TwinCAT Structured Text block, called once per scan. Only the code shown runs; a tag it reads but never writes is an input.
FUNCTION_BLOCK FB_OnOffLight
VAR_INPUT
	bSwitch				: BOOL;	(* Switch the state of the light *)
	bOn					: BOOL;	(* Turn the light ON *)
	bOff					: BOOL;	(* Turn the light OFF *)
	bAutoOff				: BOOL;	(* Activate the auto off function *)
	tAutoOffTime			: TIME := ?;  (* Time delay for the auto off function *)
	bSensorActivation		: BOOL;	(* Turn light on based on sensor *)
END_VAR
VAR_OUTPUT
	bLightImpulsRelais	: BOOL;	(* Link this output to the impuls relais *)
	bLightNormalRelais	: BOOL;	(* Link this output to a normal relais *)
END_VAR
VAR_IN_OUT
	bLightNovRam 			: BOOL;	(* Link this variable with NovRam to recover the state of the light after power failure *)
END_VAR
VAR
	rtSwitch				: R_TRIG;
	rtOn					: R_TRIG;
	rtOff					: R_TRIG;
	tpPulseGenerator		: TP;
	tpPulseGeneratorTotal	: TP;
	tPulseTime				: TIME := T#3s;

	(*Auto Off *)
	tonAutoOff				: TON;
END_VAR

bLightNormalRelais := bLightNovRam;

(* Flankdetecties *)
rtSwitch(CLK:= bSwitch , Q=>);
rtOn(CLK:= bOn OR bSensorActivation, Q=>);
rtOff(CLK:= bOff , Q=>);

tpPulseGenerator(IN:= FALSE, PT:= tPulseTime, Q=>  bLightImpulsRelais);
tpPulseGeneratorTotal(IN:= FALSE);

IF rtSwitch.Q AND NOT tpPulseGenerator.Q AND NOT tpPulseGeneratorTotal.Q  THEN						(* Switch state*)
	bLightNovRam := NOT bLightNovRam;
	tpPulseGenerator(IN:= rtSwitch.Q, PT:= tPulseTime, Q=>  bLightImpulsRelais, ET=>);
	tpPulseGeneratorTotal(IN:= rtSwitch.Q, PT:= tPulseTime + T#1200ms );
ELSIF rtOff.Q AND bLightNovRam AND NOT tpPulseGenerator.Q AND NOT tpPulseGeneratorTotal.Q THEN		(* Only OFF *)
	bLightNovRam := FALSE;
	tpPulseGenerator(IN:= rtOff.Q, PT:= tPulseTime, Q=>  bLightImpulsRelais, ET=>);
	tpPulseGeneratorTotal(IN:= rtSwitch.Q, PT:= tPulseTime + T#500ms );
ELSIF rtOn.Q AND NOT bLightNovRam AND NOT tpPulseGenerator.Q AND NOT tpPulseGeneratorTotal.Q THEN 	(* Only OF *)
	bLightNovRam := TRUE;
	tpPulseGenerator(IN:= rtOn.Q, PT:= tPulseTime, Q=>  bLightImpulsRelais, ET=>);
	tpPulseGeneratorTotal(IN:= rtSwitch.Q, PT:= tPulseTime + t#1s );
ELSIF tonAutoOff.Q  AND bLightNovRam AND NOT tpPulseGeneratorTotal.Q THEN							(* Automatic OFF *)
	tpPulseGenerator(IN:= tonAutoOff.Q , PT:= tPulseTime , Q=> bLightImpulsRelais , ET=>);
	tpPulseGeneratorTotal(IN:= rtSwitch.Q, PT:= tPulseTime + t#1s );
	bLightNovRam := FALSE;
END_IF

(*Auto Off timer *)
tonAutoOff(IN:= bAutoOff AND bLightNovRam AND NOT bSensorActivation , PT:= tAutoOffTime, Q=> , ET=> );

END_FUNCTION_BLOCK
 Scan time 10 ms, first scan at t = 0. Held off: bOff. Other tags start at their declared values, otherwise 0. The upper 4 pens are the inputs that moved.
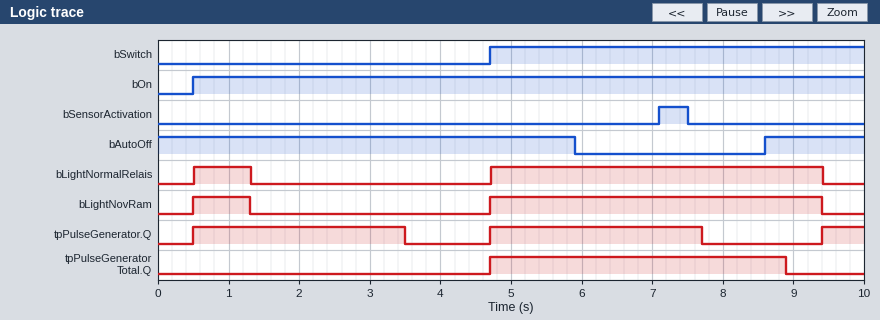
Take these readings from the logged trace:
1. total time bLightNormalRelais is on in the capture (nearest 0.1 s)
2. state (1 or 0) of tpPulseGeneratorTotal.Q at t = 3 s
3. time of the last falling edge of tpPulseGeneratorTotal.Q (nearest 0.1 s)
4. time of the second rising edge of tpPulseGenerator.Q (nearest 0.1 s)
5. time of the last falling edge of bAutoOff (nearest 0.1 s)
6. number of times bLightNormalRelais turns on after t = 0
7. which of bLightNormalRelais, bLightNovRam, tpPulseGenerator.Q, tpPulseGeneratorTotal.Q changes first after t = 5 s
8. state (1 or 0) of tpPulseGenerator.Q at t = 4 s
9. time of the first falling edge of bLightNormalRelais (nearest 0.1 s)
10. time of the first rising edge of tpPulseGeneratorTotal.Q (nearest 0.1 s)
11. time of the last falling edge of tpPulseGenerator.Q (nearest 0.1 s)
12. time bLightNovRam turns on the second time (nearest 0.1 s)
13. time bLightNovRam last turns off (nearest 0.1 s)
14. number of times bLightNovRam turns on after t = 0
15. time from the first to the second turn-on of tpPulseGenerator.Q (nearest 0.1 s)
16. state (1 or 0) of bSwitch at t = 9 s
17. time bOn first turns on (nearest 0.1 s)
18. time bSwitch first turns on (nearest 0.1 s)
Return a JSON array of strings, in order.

["5.5 s", "0", "8.9 s", "4.7 s", "5.9 s", "2", "tpPulseGenerator.Q", "0", "1.3 s", "4.7 s", "7.7 s", "4.7 s", "9.4 s", "2", "4.2 s", "1", "0.5 s", "4.7 s"]
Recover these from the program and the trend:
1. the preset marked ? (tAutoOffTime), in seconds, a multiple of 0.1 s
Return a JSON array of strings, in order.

["0.8 s"]
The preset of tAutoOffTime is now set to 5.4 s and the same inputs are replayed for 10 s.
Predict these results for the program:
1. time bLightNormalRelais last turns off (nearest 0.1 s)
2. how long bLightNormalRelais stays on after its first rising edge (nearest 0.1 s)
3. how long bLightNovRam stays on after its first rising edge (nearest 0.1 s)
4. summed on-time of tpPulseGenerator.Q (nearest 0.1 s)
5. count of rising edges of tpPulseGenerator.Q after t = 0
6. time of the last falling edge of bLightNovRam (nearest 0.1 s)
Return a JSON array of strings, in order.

["4.7 s", "4.2 s", "4.2 s", "6.0 s", "2", "4.7 s"]
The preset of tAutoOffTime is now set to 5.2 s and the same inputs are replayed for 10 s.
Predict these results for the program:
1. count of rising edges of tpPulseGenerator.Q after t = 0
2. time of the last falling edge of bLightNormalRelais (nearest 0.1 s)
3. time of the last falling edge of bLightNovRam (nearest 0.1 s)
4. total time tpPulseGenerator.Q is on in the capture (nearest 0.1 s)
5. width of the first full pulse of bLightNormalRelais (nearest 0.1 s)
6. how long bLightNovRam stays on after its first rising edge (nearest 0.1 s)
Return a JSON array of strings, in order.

["2", "4.7 s", "4.7 s", "6.0 s", "4.2 s", "4.2 s"]
